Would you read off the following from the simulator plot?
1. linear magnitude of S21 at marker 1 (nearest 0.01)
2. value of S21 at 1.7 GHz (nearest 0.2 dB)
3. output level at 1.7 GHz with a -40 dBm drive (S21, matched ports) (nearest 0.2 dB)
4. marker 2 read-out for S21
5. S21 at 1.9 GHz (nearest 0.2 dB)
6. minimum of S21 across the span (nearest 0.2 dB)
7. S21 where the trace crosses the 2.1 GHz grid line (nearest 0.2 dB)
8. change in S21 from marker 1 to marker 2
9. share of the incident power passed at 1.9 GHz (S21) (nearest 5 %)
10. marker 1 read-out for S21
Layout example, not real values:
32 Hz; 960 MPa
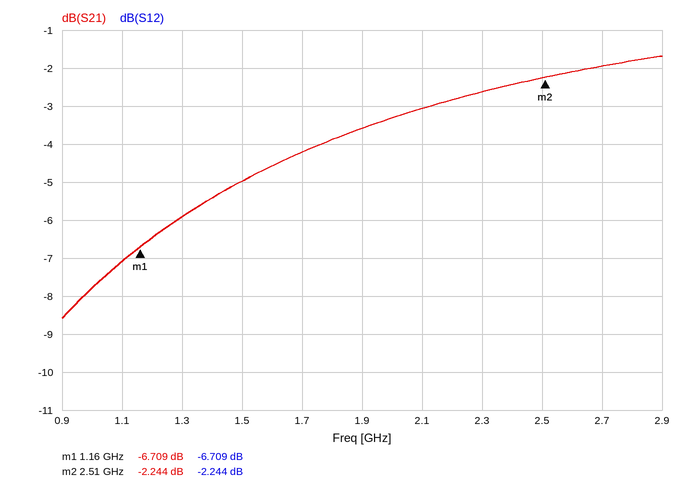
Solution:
0.46; -4.2 dB; -44.2 dBm; -2.244 dB; -3.6 dB; -8.6 dB; -3.0 dB; 4.465 dB; 45 %; -6.709 dB
